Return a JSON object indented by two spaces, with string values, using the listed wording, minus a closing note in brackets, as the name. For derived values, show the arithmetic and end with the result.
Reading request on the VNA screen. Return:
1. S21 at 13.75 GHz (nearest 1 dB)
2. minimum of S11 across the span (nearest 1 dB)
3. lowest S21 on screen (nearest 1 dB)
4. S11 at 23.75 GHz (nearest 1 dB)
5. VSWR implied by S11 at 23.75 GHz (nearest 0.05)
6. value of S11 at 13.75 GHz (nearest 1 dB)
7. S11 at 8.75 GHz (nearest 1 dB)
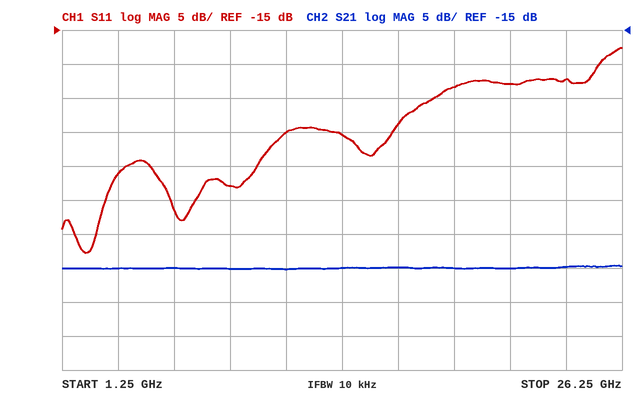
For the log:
{
  "S21 at 13.75 GHz": "-50 dB",
  "minimum of S11 across the span": "-48 dB",
  "lowest S21 on screen": "-50 dB",
  "S11 at 23.75 GHz": "-22 dB",
  "VSWR implied by S11 at 23.75 GHz": "|Γ| = 10^(-22/20) = 0.0794; VSWR = (1 + 0.0794)/(1 − 0.0794) ≈ 1.17, so 1.15 to the nearest 0.05",
  "value of S11 at 13.75 GHz": "-30 dB",
  "S11 at 8.75 GHz": "-38 dB"
}
